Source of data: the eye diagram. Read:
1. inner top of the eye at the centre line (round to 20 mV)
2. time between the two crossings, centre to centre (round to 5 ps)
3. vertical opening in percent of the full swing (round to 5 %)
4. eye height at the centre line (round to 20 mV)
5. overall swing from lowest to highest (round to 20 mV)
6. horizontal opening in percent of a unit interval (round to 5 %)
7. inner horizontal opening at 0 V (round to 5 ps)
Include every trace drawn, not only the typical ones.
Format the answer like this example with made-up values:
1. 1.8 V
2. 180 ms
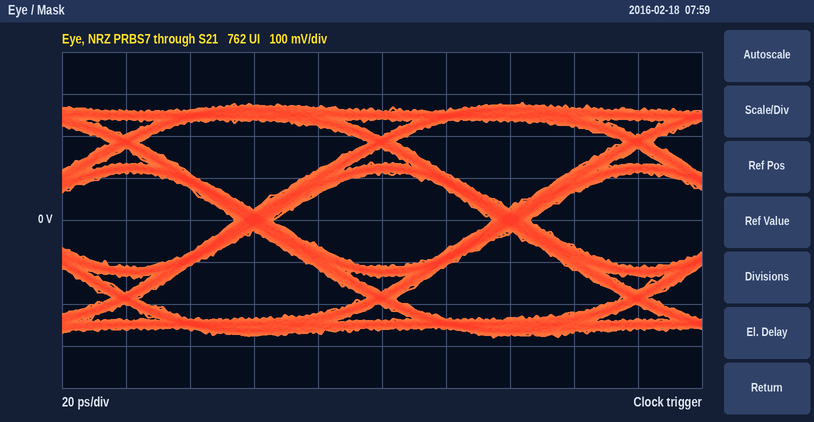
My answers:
1. 120 mV
2. 80 ps
3. 40 %
4. 220 mV
5. 560 mV
6. 85 %
7. 70 ps
